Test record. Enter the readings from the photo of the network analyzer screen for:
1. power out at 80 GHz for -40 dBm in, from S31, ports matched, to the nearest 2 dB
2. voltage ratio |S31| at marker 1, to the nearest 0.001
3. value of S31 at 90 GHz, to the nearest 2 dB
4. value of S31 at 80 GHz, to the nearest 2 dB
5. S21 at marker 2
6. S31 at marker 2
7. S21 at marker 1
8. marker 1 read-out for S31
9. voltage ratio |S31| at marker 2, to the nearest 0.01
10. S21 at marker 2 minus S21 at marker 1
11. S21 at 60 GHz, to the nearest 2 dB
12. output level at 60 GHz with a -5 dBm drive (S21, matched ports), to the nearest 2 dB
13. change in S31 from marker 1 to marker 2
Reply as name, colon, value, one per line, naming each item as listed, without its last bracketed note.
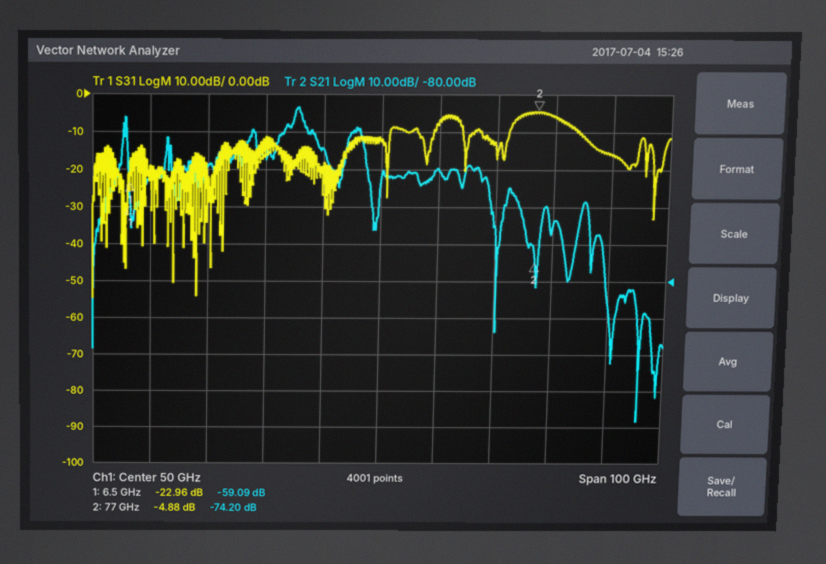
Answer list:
power out at 80 GHz for -40 dBm in, from S31, ports matched, to the nearest 2 dB: -46 dBm
voltage ratio |S31| at marker 1, to the nearest 0.001: 0.071
value of S31 at 90 GHz, to the nearest 2 dB: -16 dB
value of S31 at 80 GHz, to the nearest 2 dB: -6 dB
S21 at marker 2: -74.20 dB
S31 at marker 2: -4.88 dB
S21 at marker 1: -59.09 dB
marker 1 read-out for S31: -22.96 dB
voltage ratio |S31| at marker 2, to the nearest 0.01: 0.57
S21 at marker 2 minus S21 at marker 1: -15.11 dB
S21 at 60 GHz, to the nearest 2 dB: -50 dB
output level at 60 GHz with a -5 dBm drive (S21, matched ports), to the nearest 2 dB: -56 dBm
change in S31 from marker 1 to marker 2: 18.08 dB
